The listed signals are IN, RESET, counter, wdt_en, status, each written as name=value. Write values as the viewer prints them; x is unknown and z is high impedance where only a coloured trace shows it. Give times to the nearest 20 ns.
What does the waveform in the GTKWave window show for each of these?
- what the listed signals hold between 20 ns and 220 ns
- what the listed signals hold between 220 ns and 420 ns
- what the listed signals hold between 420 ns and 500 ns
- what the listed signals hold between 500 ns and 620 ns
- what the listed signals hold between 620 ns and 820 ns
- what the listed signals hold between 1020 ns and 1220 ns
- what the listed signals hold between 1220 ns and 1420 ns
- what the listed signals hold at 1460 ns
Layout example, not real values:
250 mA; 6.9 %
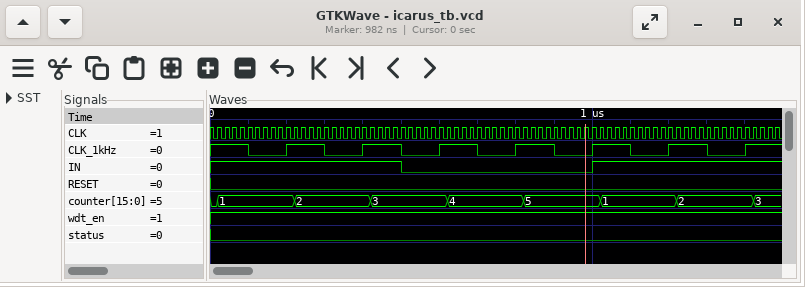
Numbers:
IN=1, RESET=0, counter=1, wdt_en=1, status=0; IN=1, RESET=0, counter=2, wdt_en=1, status=0; IN=1, RESET=0, counter=3, wdt_en=1, status=0; IN=0, RESET=0, counter=3, wdt_en=1, status=0; IN=0, RESET=0, counter=4, wdt_en=1, status=0; IN=1, RESET=0, counter=1, wdt_en=1, status=0; IN=1, RESET=0, counter=2, wdt_en=1, status=0; IN=1, RESET=0, counter=3, wdt_en=1, status=0
